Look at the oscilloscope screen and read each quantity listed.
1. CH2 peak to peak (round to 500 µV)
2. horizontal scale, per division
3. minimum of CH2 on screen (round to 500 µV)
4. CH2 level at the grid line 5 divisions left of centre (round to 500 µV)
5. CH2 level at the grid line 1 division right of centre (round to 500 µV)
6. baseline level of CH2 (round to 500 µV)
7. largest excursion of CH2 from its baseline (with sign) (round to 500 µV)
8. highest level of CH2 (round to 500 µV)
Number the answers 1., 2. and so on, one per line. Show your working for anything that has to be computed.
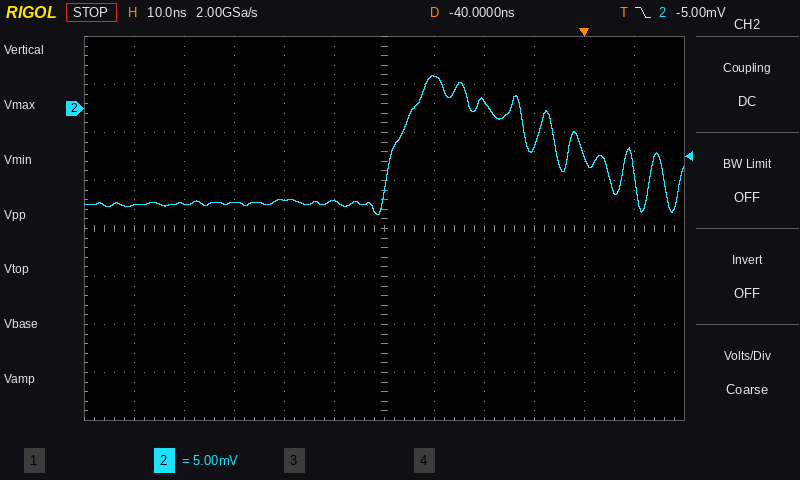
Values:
1. 3.5 mV − (-11.0 mV) = 14.5 mV
2. 10 ns
3. -11.0 mV
4. -10.0 mV
5. 3.5 mV
6. -10.0 mV
7. 3.5 mV − (-10.0 mV) = +13.5 mV
8. 3.5 mV
